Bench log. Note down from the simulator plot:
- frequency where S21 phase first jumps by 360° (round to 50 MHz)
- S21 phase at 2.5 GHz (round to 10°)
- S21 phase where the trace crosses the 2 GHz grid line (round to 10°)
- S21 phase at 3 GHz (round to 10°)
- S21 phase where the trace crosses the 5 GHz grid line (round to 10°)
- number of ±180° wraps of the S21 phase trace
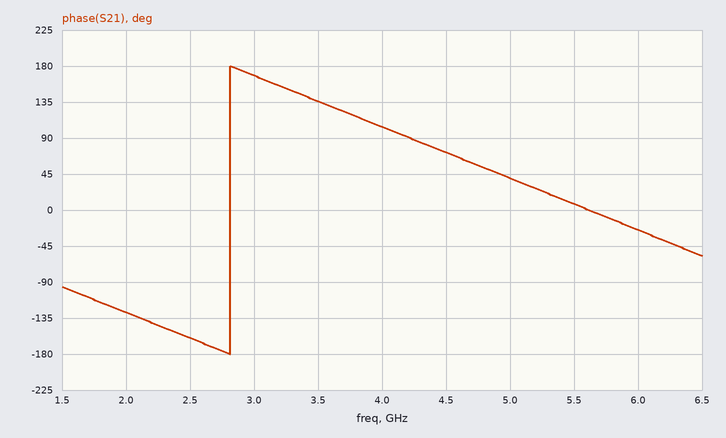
2.80 GHz
-160°
-130°
170°
40°
1
